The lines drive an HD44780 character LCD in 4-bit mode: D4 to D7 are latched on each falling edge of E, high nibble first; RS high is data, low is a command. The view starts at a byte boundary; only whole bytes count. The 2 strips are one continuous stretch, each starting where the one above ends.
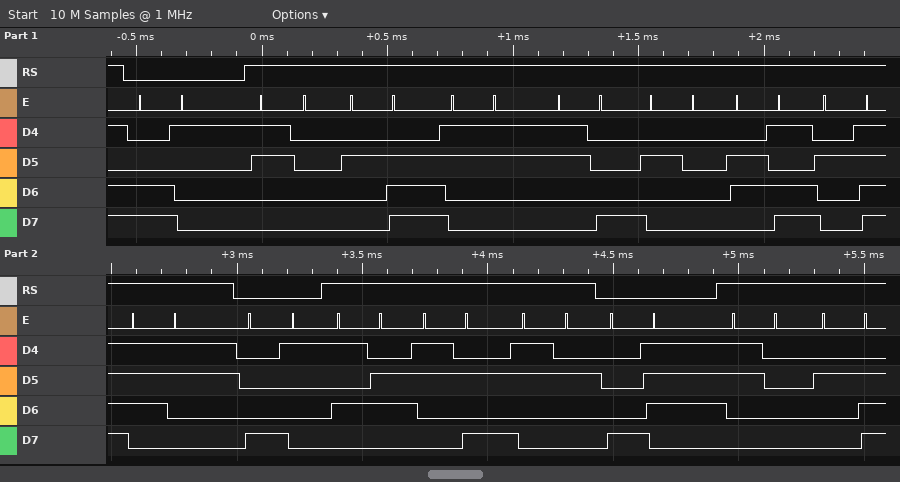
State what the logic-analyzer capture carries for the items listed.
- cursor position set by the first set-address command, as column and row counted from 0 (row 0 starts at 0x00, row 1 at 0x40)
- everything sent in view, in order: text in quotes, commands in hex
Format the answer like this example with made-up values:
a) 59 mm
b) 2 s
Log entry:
a) column 1, row 1
b) 0xC1 "0.38 m/s" 0x81 "V:2" 0x87 "0."
